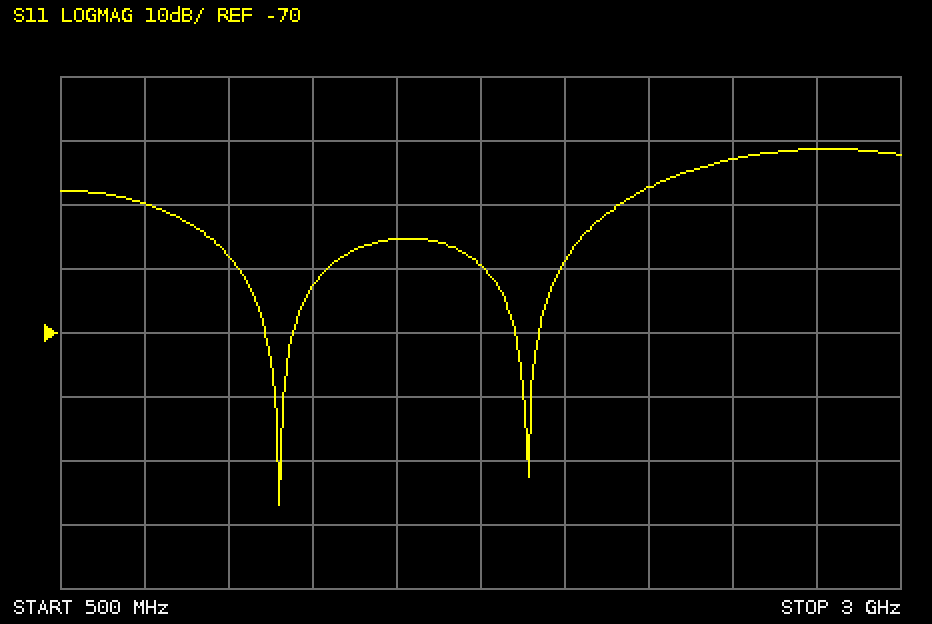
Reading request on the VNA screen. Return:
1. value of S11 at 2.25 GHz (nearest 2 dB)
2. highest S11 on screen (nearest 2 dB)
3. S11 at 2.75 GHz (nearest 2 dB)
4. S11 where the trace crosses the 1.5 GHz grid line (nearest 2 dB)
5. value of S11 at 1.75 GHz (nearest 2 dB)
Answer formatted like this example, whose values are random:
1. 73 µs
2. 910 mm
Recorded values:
1. -48 dB
2. -42 dB
3. -42 dB
4. -56 dB
5. -60 dB
